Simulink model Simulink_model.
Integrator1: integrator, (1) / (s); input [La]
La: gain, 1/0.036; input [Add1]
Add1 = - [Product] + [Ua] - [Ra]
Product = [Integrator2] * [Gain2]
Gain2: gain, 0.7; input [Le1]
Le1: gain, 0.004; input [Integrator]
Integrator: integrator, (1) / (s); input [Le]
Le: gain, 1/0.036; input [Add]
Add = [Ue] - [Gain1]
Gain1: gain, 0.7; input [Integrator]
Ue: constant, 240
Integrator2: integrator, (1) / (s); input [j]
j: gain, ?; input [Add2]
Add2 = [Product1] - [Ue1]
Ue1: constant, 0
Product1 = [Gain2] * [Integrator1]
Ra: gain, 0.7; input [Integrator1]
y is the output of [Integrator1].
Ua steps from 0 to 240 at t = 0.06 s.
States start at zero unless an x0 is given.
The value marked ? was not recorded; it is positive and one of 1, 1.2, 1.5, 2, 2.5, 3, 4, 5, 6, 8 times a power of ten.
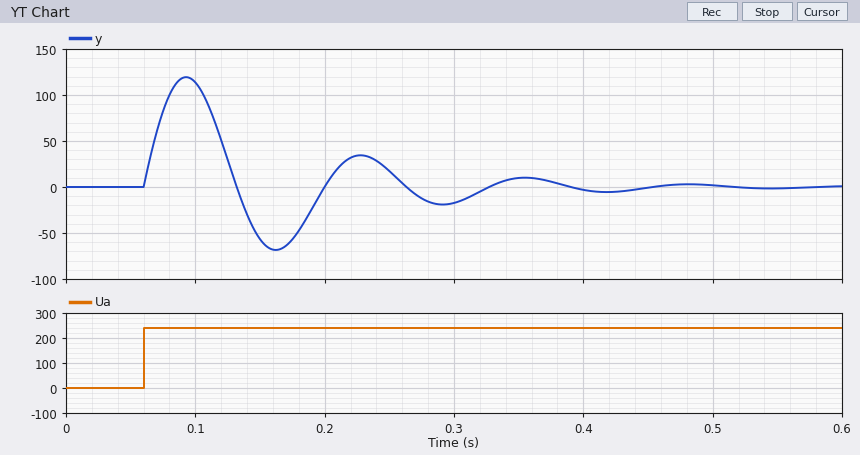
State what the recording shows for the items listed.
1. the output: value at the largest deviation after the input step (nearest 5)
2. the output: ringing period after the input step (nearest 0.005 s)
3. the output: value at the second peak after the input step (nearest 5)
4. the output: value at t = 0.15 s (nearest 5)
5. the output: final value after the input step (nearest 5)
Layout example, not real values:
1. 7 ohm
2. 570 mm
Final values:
1. 120
2. 0.135 s
3. 35
4. -55
5. 0
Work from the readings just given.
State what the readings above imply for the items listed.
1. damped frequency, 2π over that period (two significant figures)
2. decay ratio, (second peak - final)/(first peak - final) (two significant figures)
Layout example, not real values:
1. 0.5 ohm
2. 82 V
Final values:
1. 47 rad/s
2. 0.29
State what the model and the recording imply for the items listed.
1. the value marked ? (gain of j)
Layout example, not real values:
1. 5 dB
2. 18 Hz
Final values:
1. 100
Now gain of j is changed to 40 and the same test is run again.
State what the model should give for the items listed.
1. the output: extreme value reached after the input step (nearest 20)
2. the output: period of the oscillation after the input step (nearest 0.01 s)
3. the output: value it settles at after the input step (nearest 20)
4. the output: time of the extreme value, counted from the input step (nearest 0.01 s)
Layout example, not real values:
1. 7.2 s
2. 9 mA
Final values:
1. 160
2. 0.21 s
3. 0
4. 0.05 s
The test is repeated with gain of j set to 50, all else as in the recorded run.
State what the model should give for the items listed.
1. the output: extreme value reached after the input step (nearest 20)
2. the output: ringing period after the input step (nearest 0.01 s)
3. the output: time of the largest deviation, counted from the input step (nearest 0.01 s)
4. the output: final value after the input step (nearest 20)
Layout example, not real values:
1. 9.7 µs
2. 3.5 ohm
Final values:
1. 140
2. 0.19 s
3. 0.04 s
4. 0
